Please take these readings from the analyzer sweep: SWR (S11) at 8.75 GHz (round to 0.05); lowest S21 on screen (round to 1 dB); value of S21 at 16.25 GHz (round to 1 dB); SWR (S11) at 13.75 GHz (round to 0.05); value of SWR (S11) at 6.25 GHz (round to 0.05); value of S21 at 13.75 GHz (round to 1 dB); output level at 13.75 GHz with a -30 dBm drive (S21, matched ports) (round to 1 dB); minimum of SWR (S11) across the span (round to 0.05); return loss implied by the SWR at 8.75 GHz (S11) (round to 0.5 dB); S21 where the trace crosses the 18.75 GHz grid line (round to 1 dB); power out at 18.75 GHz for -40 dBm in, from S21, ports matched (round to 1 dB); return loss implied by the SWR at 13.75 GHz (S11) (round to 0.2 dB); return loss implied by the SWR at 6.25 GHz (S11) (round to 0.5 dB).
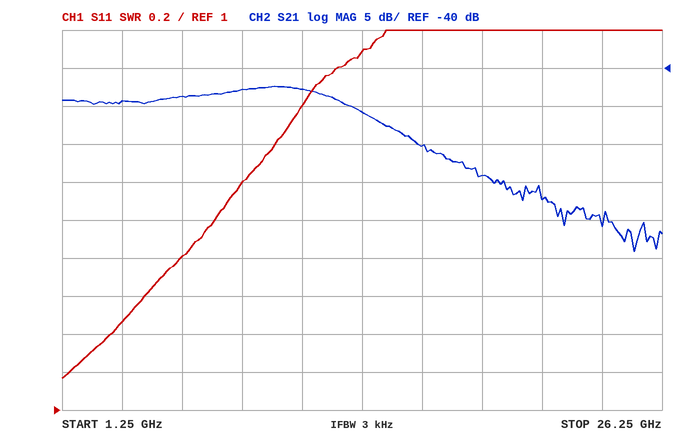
2.20
-64 dB
-50 dB
2.90
1.80
-46 dB
-76 dBm
1.15
8.5 dB
-54 dB
-94 dBm
6.2 dB
11.0 dB
